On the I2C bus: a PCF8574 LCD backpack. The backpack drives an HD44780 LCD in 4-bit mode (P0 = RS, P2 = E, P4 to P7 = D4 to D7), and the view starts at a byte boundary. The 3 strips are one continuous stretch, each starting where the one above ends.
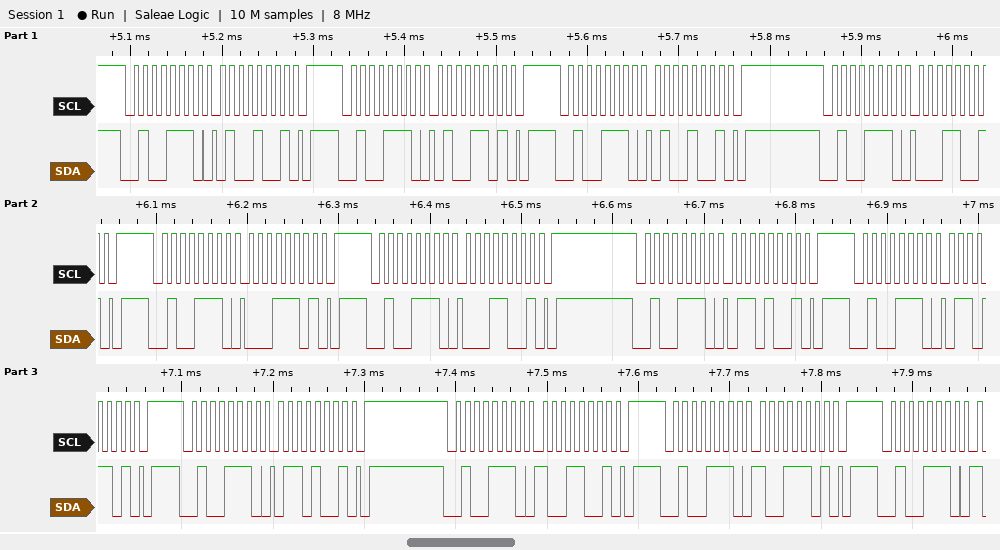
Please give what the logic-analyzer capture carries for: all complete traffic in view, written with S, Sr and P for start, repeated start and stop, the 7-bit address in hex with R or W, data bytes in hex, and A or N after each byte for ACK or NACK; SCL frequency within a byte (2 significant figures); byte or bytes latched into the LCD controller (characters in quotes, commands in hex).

S 27W A 49 A P S 27W A 4D A P S 27W A 49 A P S 27W A 19 A P S 27W A 1D A P S 27W A 19 A P S 27W A 69 A P S 27W A 6D A P S 27W A 69 A P S 27W A 99 A P S 27W A 9D A P S 27W A
100 kHz
'A'
